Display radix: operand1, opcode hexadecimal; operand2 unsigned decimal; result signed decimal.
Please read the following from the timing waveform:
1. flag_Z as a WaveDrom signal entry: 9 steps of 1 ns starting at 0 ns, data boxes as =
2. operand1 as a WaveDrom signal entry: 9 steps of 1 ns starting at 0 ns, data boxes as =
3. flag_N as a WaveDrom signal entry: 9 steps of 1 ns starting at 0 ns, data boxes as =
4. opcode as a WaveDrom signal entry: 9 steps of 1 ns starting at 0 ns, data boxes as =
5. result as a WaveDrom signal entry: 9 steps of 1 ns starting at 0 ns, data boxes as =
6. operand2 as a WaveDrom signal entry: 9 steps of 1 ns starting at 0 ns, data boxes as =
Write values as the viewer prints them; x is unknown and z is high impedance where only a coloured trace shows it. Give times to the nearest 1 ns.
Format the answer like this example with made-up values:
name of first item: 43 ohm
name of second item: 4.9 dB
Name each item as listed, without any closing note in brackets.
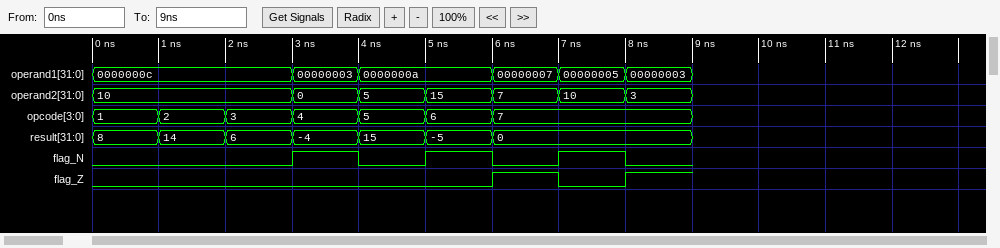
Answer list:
flag_Z as a WaveDrom signal entry: 9 steps of 1 ns starting at 0 ns, data boxes as =: {name: 'flag_Z', wave: '0.....101'}
operand1 as a WaveDrom signal entry: 9 steps of 1 ns starting at 0 ns, data boxes as =: {name: 'operand1', wave: '=..==.===', data: '0000000c 00000003 0000000a 00000007 00000005 00000003'}
flag_N as a WaveDrom signal entry: 9 steps of 1 ns starting at 0 ns, data boxes as =: {name: 'flag_N', wave: '0..101010'}
opcode as a WaveDrom signal entry: 9 steps of 1 ns starting at 0 ns, data boxes as =: {name: 'opcode', wave: '=======..', data: '1 2 3 4 5 6 7'}
result as a WaveDrom signal entry: 9 steps of 1 ns starting at 0 ns, data boxes as =: {name: 'result', wave: '=======..', data: '8 14 6 -4 15 -5 0'}
operand2 as a WaveDrom signal entry: 9 steps of 1 ns starting at 0 ns, data boxes as =: {name: 'operand2', wave: '=..======', data: '10 0 5 15 7 10 3'}
